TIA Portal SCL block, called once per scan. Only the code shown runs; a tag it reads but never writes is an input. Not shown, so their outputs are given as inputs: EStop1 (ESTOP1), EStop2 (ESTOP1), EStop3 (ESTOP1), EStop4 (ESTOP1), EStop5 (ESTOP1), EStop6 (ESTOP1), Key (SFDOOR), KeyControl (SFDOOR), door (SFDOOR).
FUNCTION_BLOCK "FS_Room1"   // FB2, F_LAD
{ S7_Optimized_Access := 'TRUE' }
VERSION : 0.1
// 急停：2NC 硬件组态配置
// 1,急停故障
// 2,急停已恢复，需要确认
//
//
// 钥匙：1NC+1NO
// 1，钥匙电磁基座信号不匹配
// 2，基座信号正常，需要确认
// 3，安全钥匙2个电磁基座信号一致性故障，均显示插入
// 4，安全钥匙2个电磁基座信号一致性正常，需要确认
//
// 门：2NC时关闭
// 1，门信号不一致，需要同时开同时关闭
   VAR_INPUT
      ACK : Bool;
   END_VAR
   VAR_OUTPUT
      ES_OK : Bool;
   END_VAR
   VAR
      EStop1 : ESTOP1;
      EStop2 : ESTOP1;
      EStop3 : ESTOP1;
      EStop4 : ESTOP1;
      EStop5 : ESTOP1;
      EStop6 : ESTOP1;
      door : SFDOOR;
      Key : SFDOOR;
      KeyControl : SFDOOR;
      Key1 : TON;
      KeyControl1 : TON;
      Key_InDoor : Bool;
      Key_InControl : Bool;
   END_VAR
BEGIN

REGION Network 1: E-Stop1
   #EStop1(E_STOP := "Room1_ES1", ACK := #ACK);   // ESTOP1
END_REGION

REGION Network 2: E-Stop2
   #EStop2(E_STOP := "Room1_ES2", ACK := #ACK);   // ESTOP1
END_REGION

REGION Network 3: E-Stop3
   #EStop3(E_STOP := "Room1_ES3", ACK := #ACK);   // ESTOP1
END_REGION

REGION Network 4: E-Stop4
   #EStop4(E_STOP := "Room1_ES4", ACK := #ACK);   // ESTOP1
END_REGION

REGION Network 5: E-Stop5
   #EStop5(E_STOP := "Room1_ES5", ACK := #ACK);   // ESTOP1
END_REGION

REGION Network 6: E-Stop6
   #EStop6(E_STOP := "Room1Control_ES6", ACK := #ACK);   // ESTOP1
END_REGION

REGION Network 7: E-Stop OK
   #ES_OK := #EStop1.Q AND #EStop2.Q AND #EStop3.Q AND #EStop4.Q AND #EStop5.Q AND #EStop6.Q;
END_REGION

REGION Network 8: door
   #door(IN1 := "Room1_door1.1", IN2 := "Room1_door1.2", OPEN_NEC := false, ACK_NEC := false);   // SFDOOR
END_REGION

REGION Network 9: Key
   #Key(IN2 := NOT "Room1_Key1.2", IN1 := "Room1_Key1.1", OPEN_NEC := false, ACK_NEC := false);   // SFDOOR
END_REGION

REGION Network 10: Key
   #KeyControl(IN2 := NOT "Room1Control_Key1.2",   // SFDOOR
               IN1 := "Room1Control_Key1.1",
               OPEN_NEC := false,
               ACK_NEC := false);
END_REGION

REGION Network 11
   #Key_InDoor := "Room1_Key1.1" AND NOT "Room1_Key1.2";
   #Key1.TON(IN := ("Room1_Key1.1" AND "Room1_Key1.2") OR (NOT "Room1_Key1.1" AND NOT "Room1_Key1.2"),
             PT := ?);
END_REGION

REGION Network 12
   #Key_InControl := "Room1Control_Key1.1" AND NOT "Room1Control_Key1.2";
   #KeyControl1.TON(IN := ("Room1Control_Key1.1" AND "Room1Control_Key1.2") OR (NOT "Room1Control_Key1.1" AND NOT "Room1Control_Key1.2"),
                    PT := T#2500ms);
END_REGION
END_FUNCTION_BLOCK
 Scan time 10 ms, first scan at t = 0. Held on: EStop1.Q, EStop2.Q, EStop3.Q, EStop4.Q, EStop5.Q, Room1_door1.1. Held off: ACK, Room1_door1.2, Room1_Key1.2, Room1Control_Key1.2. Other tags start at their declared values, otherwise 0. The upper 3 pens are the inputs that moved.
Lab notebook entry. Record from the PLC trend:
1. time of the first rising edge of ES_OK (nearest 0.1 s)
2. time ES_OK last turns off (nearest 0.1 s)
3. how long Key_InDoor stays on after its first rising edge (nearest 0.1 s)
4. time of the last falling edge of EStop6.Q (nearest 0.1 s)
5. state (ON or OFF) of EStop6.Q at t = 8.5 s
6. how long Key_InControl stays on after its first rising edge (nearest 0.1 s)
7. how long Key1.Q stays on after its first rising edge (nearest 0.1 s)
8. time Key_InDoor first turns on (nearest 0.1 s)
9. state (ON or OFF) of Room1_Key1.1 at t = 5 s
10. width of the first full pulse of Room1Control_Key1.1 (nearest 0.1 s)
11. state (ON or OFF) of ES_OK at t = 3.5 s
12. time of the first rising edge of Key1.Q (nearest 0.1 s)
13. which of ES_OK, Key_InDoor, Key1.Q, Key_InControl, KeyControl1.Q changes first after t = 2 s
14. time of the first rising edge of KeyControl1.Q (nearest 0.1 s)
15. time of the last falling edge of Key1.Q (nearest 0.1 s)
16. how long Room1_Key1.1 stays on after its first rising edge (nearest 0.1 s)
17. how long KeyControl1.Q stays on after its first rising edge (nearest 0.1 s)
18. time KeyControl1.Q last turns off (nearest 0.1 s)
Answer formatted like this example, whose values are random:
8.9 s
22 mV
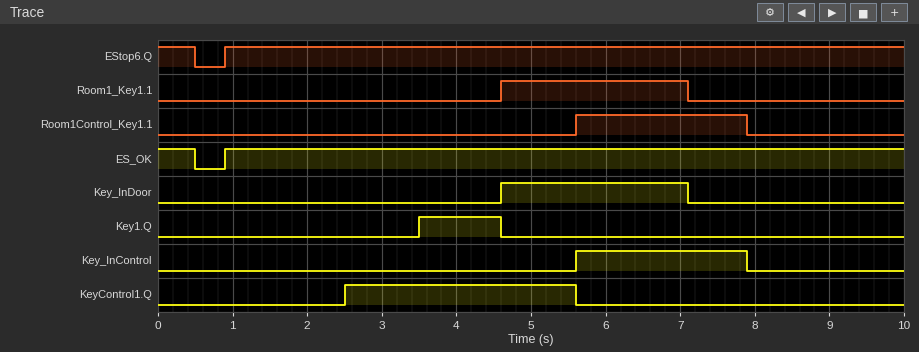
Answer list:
0.9 s
0.5 s
2.5 s
0.5 s
ON
2.3 s
1.1 s
4.6 s
ON
2.3 s
ON
3.5 s
KeyControl1.Q
2.5 s
4.6 s
2.5 s
3.1 s
5.6 s
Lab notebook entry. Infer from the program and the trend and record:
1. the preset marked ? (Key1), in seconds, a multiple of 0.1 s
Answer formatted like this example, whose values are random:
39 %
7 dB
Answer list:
3.5 s
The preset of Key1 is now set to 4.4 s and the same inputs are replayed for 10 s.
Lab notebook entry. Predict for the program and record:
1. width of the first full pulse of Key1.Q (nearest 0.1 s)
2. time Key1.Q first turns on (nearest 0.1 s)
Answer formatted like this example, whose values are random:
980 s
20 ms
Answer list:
0.2 s
4.4 s
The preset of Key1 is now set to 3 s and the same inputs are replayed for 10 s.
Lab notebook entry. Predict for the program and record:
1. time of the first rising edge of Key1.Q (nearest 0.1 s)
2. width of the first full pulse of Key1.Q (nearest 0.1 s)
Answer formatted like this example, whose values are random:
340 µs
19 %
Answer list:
3.0 s
1.6 s
